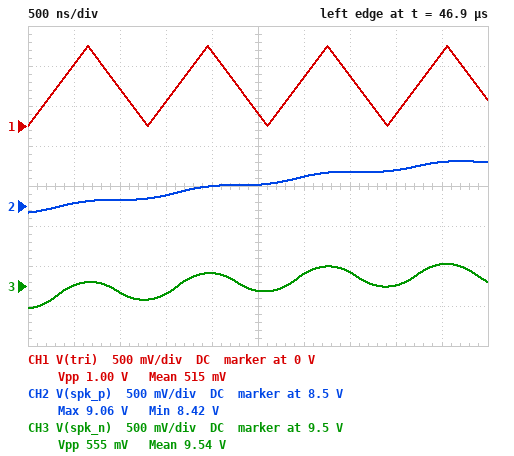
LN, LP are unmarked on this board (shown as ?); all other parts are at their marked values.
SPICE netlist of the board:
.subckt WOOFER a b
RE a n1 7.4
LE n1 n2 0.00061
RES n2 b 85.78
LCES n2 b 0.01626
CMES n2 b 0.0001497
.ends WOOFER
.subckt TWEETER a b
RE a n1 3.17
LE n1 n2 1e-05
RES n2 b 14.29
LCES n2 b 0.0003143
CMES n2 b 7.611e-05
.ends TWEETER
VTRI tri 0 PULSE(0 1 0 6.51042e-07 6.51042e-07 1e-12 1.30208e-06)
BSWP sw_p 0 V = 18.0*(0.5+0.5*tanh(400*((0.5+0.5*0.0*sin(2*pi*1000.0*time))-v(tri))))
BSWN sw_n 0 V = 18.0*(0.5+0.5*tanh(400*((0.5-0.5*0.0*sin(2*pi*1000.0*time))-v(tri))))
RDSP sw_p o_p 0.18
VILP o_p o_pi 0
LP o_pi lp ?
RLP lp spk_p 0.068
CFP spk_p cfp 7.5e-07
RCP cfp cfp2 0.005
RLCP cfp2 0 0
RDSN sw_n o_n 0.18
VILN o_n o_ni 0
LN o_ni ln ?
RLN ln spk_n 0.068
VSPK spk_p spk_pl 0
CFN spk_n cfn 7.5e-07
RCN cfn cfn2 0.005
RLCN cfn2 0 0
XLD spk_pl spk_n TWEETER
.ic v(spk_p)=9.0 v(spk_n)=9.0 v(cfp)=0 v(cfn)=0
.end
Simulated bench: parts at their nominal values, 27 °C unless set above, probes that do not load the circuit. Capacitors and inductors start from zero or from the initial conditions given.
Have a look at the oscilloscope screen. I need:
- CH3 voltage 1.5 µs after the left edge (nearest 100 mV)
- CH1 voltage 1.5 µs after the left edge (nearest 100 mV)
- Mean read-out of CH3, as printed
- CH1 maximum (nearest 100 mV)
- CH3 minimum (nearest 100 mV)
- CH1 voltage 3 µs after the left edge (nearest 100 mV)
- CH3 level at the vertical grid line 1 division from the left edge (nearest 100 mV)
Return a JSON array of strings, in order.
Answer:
["9.4 V", "300 mV", "9.54 V", "1.0 V", "9.2 V", "600 mV", "9.5 V"]
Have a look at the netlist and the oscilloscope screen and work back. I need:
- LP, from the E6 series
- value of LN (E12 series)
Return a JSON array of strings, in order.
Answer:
["22 µH", "4.7 µH"]
